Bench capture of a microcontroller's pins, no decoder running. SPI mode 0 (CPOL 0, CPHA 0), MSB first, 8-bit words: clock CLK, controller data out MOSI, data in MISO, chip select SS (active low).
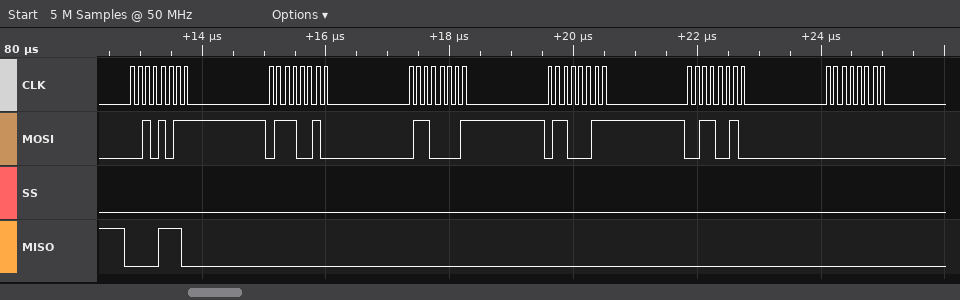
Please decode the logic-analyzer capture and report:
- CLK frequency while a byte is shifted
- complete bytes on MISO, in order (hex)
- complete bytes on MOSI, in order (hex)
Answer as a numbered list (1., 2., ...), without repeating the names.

1. 8 MHz
2. 0E 00 00 00 00 00
3. 2B 72 61 63 32 00
